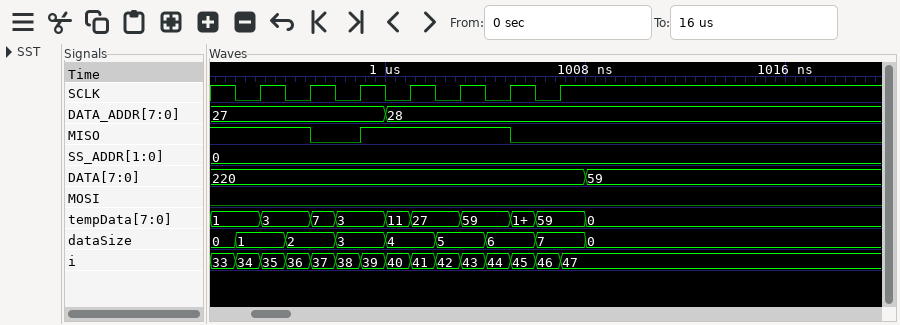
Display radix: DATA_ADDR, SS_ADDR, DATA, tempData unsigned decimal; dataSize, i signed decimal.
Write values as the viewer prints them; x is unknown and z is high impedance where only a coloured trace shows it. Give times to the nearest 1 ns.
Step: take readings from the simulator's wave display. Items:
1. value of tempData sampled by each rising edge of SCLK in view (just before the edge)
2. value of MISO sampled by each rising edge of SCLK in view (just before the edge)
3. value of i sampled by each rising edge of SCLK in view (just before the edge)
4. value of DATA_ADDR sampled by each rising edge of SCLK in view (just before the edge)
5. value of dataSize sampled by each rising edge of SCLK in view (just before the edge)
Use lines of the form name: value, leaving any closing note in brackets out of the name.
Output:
value of tempData sampled by each rising edge of SCLK in view: 1, 3, 3, 11, 27, 59, 59
value of MISO sampled by each rising edge of SCLK in view: 1 1 0 1 1 1 0
value of i sampled by each rising edge of SCLK in view: 34, 36, 38, 40, 42, 44, 46
value of DATA_ADDR sampled by each rising edge of SCLK in view: 27, 27, 27, 28, 28, 28, 28
value of dataSize sampled by each rising edge of SCLK in view: 1, 2, 3, 4, 5, 6, 7
